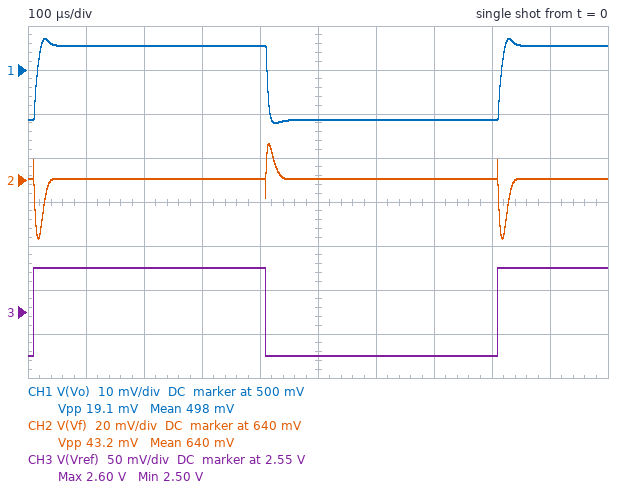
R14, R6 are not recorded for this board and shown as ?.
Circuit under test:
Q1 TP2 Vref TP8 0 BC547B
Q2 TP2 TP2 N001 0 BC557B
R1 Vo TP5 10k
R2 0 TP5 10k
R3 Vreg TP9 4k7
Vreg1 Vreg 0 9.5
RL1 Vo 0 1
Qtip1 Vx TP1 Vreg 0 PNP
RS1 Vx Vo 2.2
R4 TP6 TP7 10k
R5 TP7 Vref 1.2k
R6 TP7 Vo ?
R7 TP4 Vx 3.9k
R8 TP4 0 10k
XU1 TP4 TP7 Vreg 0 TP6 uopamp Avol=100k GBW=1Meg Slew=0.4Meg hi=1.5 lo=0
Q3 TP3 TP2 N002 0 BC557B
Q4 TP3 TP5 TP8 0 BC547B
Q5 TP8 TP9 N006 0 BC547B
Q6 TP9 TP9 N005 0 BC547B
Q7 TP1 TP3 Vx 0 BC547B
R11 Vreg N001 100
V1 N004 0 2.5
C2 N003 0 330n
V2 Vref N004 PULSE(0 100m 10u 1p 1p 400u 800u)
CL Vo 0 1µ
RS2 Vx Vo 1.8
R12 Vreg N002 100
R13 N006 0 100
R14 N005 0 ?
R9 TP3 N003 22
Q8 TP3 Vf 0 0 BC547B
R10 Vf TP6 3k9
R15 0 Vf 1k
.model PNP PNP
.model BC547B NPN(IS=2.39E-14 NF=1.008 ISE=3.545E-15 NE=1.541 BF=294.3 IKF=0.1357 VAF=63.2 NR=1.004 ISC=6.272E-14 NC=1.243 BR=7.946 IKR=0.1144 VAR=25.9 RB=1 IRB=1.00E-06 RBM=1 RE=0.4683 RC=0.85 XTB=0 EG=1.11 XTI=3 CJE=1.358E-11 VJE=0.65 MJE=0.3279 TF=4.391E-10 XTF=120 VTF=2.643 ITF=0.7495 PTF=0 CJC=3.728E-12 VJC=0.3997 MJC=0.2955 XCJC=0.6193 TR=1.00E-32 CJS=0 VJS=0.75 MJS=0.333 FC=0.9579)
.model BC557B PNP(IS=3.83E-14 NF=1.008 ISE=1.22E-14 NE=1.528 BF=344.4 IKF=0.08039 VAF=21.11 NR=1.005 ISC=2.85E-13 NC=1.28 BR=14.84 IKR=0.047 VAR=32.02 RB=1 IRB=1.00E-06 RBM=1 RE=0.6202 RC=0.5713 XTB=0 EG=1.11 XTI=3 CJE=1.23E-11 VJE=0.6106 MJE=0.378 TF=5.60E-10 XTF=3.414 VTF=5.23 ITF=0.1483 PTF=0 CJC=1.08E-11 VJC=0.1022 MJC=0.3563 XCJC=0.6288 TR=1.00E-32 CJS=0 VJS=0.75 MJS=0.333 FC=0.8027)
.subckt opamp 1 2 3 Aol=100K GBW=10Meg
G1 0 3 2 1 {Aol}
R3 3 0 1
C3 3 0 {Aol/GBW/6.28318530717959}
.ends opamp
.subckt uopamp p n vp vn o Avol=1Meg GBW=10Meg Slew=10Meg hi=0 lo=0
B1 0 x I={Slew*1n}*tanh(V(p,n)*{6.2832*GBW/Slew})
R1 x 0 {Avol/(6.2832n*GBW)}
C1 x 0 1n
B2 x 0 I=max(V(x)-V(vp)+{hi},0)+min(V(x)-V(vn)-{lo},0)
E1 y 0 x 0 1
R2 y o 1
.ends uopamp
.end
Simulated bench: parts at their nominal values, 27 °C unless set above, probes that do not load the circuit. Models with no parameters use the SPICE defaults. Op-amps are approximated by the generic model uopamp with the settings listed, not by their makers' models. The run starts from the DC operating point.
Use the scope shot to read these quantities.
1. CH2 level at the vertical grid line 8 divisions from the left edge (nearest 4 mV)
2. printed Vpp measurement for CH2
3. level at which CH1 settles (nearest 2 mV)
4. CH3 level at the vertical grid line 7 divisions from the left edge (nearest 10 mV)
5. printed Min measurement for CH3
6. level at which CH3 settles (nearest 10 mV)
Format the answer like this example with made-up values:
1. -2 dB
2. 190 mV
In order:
1. 640 mV
2. 43.2 mV
3. 506 mV
4. 2.50 V
5. 2.50 V
6. 2.60 V
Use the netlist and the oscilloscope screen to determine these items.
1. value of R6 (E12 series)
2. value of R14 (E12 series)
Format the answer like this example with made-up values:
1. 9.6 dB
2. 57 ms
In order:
1. 120 Ω
2. 47 Ω
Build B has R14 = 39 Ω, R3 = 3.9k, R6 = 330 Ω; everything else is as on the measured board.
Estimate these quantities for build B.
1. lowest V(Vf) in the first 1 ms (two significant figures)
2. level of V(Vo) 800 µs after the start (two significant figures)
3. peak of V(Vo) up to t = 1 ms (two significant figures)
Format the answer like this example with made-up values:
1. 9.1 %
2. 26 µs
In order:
1. 580 mV
2. 910 mV
3. 940 mV
